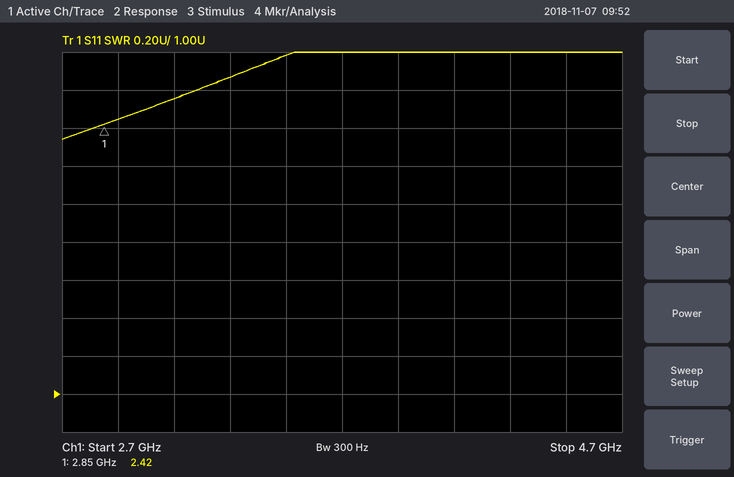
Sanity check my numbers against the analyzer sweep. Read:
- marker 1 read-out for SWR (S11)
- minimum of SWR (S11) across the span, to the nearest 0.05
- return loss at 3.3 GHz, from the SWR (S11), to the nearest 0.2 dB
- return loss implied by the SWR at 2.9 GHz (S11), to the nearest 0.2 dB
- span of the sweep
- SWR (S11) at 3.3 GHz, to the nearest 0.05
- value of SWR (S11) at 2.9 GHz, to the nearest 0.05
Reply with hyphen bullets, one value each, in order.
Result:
- 2.42
- 2.35
- 6.8 dB
- 7.6 dB
- 2 GHz
- 2.65
- 2.45
